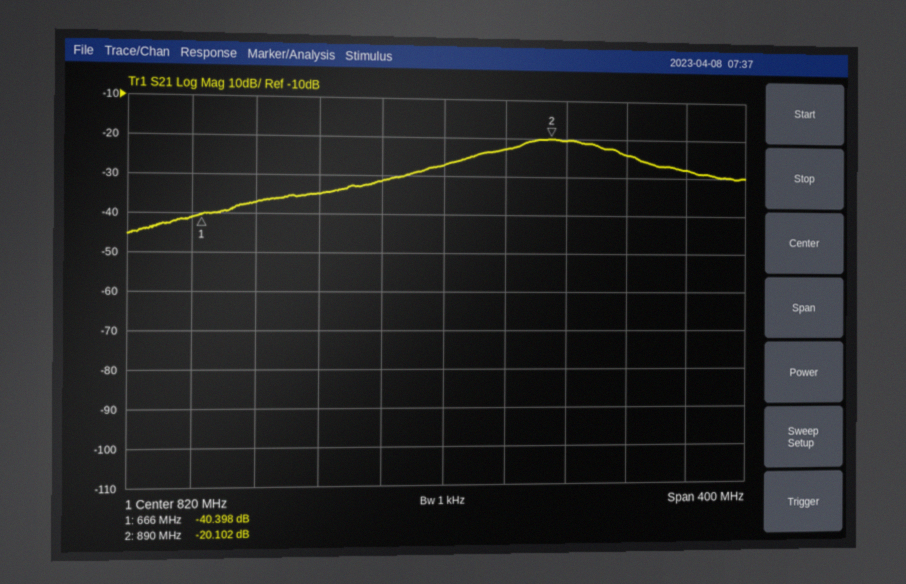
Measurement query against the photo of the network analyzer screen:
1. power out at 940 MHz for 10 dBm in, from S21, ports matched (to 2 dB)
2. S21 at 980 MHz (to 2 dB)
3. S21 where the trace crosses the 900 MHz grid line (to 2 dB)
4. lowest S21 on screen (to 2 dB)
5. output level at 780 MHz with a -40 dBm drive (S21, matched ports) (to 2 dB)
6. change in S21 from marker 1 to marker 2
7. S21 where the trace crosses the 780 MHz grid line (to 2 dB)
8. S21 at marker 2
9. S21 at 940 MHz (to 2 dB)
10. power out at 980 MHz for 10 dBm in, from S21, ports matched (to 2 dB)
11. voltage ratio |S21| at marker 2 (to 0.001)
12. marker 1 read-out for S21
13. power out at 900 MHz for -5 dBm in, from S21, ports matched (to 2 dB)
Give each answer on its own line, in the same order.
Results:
-14 dBm
-28 dB
-20 dB
-46 dB
-72 dBm
20.296 dB
-32 dB
-20.102 dB
-24 dB
-18 dBm
0.099
-40.398 dB
-26 dBm
